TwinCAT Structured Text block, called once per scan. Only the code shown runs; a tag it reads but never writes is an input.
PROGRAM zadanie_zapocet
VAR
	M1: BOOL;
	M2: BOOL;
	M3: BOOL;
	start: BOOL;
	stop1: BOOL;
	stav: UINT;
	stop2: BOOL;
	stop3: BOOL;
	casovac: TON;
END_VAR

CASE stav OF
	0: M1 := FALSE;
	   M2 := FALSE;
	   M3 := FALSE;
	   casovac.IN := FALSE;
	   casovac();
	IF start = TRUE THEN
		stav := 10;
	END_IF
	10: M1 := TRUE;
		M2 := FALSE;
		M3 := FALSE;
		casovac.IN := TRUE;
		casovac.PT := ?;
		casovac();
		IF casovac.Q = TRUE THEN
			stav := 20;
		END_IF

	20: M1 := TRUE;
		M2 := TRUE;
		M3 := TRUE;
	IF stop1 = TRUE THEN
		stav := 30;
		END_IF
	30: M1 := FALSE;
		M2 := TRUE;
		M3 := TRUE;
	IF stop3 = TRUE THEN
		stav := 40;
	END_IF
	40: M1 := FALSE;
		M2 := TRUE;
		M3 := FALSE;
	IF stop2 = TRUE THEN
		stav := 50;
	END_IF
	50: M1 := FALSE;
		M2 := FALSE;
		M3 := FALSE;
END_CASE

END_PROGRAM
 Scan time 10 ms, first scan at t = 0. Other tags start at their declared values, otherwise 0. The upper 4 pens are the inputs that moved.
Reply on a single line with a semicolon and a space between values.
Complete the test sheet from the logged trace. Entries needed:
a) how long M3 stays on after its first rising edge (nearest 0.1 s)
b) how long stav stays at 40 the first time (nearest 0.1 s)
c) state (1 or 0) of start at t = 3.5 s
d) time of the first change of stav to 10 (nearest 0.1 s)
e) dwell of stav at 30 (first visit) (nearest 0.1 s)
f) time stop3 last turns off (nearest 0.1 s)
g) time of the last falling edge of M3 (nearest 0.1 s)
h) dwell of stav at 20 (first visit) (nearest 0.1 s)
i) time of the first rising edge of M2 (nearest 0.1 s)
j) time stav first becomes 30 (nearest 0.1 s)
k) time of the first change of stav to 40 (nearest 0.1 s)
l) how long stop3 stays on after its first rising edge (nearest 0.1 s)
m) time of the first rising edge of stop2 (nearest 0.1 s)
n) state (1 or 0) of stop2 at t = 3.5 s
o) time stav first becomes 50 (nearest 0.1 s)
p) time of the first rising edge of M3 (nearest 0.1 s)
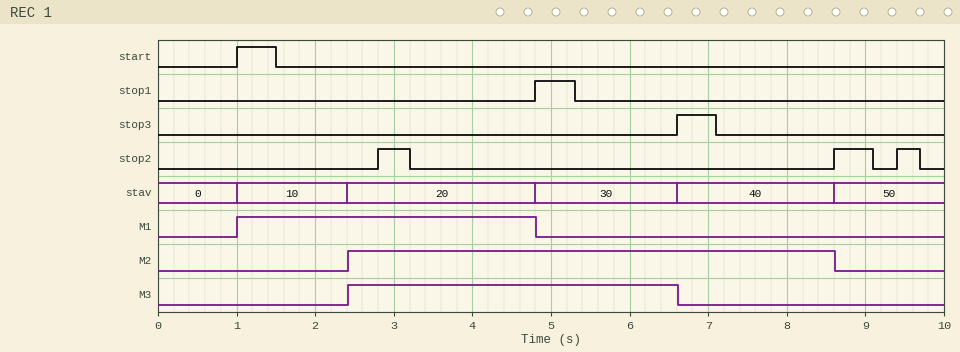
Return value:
4.2 s; 2.0 s; 0; 1.0 s; 1.8 s; 7.1 s; 6.6 s; 2.4 s; 2.4 s; 4.8 s; 6.6 s; 0.5 s; 2.8 s; 0; 8.6 s; 2.4 s
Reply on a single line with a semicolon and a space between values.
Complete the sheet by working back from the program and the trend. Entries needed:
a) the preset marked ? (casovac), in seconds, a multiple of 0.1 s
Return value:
1.4 s
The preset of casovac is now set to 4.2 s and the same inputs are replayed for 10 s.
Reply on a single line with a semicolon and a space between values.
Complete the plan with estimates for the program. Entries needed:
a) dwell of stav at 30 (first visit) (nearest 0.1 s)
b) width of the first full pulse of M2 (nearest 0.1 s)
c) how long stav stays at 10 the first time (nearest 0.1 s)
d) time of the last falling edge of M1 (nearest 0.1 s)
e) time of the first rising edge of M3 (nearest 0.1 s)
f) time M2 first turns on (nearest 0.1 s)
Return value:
1.4 s; 3.4 s; 4.2 s; 5.2 s; 5.2 s; 5.2 s
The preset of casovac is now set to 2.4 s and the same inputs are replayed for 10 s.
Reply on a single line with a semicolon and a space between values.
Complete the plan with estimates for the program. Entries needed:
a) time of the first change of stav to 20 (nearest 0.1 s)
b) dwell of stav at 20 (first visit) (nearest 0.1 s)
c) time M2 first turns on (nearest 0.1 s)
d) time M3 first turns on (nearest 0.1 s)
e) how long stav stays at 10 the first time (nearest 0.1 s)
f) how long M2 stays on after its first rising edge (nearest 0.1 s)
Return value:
3.4 s; 1.4 s; 3.4 s; 3.4 s; 2.4 s; 5.2 s
